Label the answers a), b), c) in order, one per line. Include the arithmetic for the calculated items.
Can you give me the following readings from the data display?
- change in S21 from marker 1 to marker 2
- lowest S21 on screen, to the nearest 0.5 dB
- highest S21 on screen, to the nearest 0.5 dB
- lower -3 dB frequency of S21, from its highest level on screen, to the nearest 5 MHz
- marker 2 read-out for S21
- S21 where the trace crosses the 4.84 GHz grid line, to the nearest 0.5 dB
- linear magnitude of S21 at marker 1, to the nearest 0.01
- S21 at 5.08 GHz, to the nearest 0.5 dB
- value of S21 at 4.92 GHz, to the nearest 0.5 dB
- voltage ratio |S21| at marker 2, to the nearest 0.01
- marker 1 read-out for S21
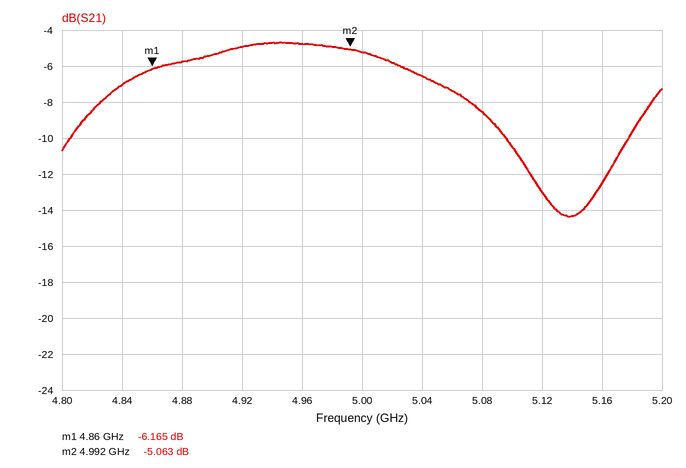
a) -5.063 − (-6.165) = 1.102 dB
b) -14.5 dB
c) -4.5 dB
d) 4.830 GHz
e) -5.063 dB
f) -7.0 dB
g) 10^(-6.165/20) ≈ 0.49
h) -8.5 dB
i) -5.0 dB
j) 10^(-5.063/20) ≈ 0.56
k) -6.165 dB
